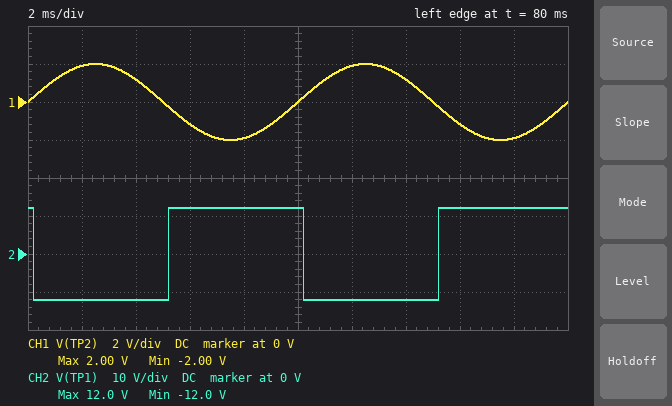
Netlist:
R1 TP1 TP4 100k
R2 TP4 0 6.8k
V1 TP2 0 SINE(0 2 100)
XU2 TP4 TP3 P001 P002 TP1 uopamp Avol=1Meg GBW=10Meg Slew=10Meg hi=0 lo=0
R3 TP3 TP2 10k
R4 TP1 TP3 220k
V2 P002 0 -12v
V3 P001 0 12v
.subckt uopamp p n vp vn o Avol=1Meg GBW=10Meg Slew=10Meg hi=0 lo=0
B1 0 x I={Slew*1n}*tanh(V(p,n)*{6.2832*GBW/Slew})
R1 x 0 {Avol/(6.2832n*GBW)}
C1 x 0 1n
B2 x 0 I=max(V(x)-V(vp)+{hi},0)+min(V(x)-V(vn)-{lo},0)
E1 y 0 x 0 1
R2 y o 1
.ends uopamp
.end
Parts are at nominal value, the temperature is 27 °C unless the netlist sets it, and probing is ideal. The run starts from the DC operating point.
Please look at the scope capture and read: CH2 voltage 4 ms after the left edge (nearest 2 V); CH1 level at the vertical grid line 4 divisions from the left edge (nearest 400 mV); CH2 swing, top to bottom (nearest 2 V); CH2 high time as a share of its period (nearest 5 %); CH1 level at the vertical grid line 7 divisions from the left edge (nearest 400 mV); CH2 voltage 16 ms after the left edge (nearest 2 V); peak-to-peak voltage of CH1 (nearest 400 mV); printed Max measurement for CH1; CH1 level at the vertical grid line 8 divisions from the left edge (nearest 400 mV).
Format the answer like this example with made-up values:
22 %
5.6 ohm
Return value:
-12 V
-2.0 V
24 V
50 %
1.2 V
12 V
4.0 V
2.00 V
-1.2 V
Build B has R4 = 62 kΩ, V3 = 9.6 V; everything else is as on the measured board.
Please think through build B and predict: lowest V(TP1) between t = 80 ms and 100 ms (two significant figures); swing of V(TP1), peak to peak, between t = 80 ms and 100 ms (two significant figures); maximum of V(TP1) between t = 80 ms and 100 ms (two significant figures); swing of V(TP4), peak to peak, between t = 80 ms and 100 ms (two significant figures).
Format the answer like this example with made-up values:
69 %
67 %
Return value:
-12 V
22 V
9.6 V
1.4 V
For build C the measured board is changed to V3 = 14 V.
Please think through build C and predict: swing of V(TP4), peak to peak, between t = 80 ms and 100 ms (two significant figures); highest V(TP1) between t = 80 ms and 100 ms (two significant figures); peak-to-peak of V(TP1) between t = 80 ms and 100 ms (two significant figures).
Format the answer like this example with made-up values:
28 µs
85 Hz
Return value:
1.7 V
14 V
26 V
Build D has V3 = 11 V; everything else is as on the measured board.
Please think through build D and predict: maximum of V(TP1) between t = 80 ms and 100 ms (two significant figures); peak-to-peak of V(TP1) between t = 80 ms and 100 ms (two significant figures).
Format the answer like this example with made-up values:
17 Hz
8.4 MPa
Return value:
11 V
23 V
